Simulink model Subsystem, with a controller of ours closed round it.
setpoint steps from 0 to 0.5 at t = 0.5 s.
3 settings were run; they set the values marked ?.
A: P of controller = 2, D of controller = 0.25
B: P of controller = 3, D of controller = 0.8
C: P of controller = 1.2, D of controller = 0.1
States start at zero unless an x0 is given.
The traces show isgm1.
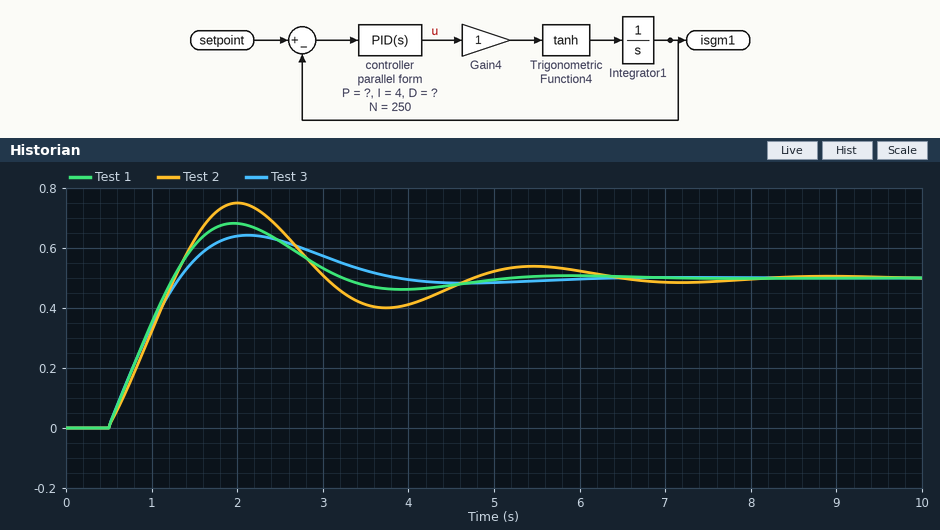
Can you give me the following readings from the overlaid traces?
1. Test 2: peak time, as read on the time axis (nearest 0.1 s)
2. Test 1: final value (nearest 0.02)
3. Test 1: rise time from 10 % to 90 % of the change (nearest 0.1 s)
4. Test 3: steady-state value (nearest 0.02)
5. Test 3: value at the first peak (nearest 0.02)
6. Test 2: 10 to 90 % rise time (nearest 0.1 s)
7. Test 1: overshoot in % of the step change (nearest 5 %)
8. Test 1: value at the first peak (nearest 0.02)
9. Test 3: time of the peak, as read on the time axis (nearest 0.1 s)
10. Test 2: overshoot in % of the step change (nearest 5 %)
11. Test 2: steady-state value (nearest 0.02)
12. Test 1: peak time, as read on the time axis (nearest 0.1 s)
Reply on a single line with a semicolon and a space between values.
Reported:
2.0 s; 0.50; 0.6 s; 0.50; 0.64; 0.6 s; 35 %; 0.68; 2.1 s; 50 %; 0.50; 2.0 s
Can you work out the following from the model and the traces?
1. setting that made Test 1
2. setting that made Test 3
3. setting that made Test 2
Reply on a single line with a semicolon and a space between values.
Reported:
A; B; C
